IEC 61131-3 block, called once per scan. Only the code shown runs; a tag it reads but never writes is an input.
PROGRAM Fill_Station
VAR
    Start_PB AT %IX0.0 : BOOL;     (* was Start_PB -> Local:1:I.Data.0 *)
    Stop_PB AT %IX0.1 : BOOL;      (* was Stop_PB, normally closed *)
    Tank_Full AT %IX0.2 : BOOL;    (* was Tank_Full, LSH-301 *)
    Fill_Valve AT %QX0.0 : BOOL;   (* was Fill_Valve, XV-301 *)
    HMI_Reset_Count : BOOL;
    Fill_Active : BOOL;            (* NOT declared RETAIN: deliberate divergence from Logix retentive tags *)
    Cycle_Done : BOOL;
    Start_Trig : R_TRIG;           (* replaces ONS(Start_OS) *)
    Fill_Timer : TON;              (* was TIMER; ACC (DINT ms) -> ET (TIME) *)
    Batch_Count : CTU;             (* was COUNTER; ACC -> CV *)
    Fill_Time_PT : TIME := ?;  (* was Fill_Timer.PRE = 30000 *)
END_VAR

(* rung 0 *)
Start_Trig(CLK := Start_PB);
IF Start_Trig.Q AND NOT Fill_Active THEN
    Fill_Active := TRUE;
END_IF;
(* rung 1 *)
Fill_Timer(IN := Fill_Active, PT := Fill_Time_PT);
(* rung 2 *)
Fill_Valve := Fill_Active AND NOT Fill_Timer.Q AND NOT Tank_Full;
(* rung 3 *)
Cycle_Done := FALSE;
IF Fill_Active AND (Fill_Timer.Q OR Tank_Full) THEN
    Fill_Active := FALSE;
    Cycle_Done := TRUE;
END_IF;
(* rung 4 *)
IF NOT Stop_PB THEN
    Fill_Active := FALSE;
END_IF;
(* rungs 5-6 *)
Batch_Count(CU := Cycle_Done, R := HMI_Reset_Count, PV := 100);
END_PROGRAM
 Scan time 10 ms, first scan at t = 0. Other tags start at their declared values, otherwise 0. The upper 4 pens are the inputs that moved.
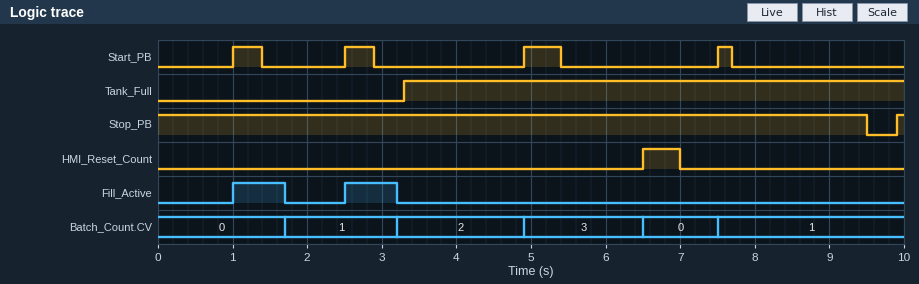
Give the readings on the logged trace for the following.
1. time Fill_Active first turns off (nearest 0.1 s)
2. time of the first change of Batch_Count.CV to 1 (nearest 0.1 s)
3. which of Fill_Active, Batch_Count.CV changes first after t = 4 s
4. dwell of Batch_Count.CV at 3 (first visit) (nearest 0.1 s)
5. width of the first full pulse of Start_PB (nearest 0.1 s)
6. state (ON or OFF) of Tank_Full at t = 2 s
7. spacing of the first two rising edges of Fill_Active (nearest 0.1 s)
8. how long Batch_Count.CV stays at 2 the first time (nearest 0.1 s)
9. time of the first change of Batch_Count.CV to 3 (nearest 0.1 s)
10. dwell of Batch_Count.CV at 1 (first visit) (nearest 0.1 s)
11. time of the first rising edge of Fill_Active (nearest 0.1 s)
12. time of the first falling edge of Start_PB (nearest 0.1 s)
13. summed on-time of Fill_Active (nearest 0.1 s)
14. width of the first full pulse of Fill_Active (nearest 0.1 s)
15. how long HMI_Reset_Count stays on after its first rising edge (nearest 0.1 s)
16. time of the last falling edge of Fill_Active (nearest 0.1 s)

1.7 s
1.7 s
Batch_Count.CV
1.6 s
0.4 s
OFF
1.5 s
1.7 s
4.9 s
1.5 s
1.0 s
1.4 s
1.4 s
0.7 s
0.5 s
3.2 s
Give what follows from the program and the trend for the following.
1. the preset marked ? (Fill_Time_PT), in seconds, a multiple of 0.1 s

0.7 s
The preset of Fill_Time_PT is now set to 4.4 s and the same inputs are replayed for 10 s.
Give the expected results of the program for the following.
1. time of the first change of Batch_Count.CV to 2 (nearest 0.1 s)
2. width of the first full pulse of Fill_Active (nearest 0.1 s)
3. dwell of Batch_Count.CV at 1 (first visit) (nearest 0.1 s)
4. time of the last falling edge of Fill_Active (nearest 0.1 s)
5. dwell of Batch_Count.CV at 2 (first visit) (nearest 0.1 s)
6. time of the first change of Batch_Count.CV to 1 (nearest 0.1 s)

4.9 s
2.3 s
1.6 s
3.3 s
1.6 s
3.3 s
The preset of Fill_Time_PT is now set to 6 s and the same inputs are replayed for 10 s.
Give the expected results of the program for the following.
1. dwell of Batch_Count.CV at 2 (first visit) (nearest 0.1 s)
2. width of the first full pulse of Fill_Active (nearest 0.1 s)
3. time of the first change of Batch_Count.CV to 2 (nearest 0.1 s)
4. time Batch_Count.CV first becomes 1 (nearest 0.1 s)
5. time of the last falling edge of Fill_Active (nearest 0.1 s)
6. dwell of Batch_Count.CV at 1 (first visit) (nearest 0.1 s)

1.6 s
2.3 s
4.9 s
3.3 s
3.3 s
1.6 s
